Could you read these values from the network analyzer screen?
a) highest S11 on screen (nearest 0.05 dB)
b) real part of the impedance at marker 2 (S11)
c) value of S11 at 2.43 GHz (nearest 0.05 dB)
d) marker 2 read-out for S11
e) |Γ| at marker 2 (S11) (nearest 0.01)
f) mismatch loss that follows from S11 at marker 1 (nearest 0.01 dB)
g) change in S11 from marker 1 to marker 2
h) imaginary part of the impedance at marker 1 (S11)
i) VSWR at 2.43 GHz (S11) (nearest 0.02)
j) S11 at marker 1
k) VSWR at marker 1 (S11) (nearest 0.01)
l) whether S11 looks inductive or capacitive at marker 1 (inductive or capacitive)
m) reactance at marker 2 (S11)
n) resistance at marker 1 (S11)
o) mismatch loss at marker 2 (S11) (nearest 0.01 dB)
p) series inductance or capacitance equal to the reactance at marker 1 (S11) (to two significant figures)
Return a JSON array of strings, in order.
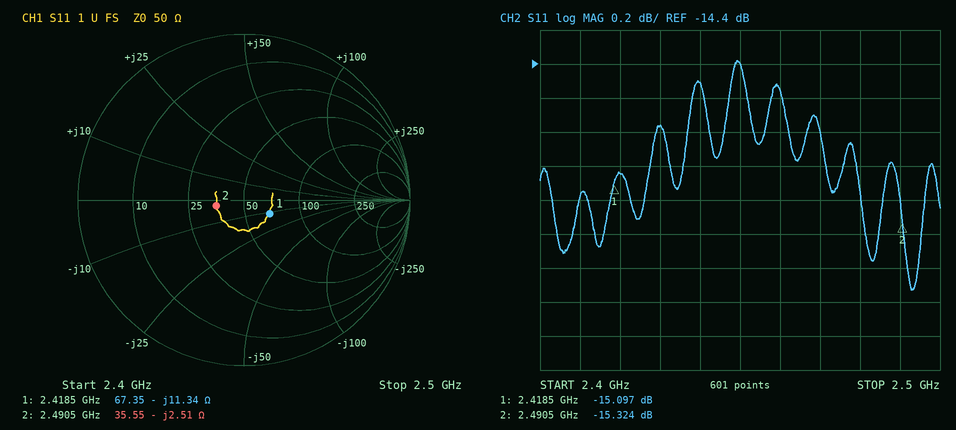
["-14.40 dB", "35.55 Ω", "-14.75 dB", "-15.324 dB", "0.17", "0.14 dB", "-0.227 dB", "-11.34 Ω", "1.44", "-15.097 dB", "1.43", "capacitive", "-2.51 Ω", "67.35 Ω", "0.13 dB", "5.8 pF"]
